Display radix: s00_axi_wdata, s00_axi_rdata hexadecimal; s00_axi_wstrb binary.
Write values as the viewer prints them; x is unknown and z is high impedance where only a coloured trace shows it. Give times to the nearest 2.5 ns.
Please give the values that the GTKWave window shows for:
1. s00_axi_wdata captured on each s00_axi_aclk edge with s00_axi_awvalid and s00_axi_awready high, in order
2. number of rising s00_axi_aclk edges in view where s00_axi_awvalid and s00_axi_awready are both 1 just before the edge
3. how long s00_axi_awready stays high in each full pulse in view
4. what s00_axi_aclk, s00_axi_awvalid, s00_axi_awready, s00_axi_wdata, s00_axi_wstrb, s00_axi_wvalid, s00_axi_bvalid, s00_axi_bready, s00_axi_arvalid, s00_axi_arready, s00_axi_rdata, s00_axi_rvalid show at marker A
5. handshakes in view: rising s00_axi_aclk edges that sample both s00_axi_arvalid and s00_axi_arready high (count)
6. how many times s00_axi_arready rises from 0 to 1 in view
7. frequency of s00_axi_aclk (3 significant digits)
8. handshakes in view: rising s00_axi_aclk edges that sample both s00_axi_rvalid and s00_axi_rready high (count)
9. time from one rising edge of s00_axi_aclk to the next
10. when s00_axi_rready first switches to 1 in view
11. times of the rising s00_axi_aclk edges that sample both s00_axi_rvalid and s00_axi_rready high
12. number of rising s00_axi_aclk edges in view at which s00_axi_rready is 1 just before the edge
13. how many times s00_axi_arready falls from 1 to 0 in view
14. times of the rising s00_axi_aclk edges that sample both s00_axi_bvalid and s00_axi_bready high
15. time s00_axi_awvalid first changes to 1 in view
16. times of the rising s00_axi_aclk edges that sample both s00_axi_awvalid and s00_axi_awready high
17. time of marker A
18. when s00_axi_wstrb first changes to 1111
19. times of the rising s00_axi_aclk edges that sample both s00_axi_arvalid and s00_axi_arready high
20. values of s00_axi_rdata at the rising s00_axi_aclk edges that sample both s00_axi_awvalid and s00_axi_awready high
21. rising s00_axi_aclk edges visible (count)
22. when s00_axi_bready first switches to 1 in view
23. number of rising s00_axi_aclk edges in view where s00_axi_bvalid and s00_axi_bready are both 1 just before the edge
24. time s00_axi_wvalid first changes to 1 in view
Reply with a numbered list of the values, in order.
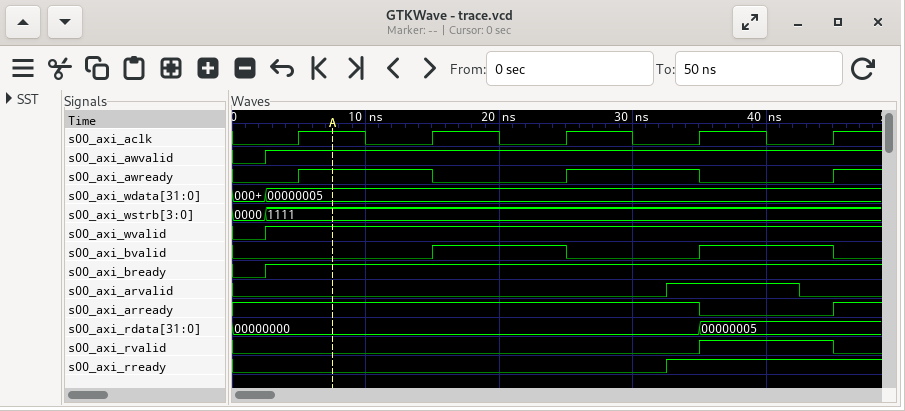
1. 00000005, 00000005
2. 2
3. 10 ns, 10 ns
4. s00_axi_aclk=1, s00_axi_awvalid=1, s00_axi_awready=1, s00_axi_wdata=00000005, s00_axi_wstrb=1111, s00_axi_wvalid=1, s00_axi_bvalid=0, s00_axi_bready=1, s00_axi_arvalid=0, s00_axi_arready=1, s00_axi_rdata=00000000, s00_axi_rvalid=0
5. 1
6. 1
7. 100 MHz
8. 1
9. 10 ns
10. 32.5 ns
11. 45 ns
12. 2
13. 1
14. 25 ns, 45 ns
15. 2.5 ns
16. 15 ns, 35 ns
17. 7.5 ns
18. 2.5 ns
19. 35 ns
20. 00000000, 00000000
21. 5
22. 2.5 ns
23. 2
24. 2.5 ns
